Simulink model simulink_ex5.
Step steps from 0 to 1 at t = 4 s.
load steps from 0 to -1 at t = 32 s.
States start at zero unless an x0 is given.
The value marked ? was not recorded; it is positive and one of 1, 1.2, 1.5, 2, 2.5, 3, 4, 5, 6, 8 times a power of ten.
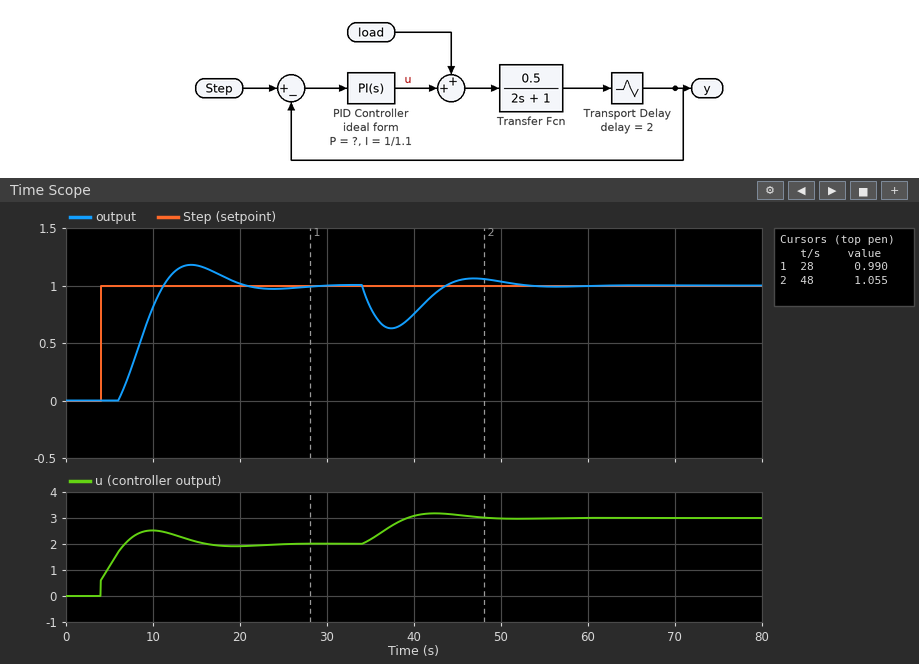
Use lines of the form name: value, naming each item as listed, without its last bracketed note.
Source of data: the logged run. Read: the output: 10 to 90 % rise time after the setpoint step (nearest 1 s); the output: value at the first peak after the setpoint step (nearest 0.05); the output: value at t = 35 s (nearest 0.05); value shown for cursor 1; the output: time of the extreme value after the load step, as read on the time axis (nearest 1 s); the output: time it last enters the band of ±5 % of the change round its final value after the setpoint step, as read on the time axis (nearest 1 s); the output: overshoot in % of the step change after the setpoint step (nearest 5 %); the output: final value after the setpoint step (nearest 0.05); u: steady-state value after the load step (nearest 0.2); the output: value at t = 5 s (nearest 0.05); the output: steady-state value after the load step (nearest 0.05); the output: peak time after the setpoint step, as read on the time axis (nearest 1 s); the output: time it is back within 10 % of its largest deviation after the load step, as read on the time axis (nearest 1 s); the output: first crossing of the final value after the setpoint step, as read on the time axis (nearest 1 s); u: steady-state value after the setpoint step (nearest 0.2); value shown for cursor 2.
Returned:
the output: 10 to 90 % rise time after the setpoint step: 4 s
the output: value at the first peak after the setpoint step: 1.20
the output: value at t = 35 s: 0.80
value shown for cursor 1: 0.990
the output: time of the extreme value after the load step, as read on the time axis: 37 s
the output: time it last enters the band of ±5 % of the change round its final value after the setpoint step, as read on the time axis: 19 s
the output: overshoot in % of the step change after the setpoint step: 20 %
the output: final value after the setpoint step: 1.00
u: steady-state value after the load step: 3.0
the output: value at t = 5 s: 0.00
the output: steady-state value after the load step: 1.00
the output: peak time after the setpoint step, as read on the time axis: 14 s
the output: time it is back within 10 % of its largest deviation after the load step, as read on the time axis: 50 s
the output: first crossing of the final value after the setpoint step, as read on the time axis: 11 s
u: steady-state value after the setpoint step: 2.0
value shown for cursor 2: 1.055
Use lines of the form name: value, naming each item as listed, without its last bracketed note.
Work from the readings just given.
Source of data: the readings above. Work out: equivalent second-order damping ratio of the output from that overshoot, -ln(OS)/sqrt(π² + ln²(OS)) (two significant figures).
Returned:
equivalent second-order damping ratio of the output from that overshoot, -ln(OS)/sqrt(π² + ln²(OS)): 0.46
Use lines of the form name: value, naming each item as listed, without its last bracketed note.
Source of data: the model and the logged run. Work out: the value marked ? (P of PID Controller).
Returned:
the value marked ?: 0.6
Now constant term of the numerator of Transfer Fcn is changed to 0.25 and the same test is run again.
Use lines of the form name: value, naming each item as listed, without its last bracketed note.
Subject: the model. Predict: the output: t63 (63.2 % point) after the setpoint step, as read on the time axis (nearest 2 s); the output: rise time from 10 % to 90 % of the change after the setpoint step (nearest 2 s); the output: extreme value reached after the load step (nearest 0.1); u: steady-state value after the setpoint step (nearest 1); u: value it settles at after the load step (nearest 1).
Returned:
the output: t63 (63.2 % point) after the setpoint step, as read on the time axis: 12 s
the output: rise time from 10 % to 90 % of the change after the setpoint step: 10 s
the output: extreme value reached after the load step: 0.8
u: steady-state value after the setpoint step: 4
u: value it settles at after the load step: 5
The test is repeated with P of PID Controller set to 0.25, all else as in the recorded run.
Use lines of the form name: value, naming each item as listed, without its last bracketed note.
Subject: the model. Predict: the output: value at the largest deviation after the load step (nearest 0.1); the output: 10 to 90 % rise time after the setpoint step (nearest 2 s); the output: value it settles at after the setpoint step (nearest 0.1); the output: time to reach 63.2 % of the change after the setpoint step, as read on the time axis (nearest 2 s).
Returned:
the output: value at the largest deviation after the load step: 0.6
the output: 10 to 90 % rise time after the setpoint step: 12 s
the output: value it settles at after the setpoint step: 1.0
the output: time to reach 63.2 % of the change after the setpoint step, as read on the time axis: 14 s
